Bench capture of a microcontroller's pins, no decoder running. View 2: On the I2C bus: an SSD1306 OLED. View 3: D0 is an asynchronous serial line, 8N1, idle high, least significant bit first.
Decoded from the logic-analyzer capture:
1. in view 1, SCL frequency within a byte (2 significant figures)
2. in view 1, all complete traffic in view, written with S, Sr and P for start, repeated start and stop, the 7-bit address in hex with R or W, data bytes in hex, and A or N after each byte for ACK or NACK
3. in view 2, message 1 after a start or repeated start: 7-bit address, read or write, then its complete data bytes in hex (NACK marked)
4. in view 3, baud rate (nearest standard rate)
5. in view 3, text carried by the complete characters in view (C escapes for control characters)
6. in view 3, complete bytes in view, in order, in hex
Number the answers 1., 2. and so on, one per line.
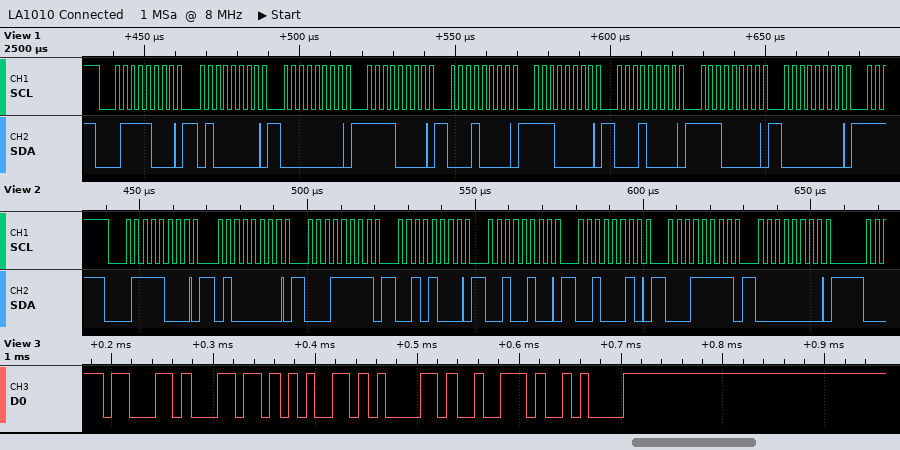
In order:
1. 400 kHz
2. S 3CW A 40 A 00 A F0 A 10 A E0 A 10 A E0 A 00 A
3. 0x3C write: 40 1F 28 24 22 1F 00
4. 115200 baud
5. "clear\n"
6. 0x63 0x6C 0x65 0x61 0x72 0x0A
